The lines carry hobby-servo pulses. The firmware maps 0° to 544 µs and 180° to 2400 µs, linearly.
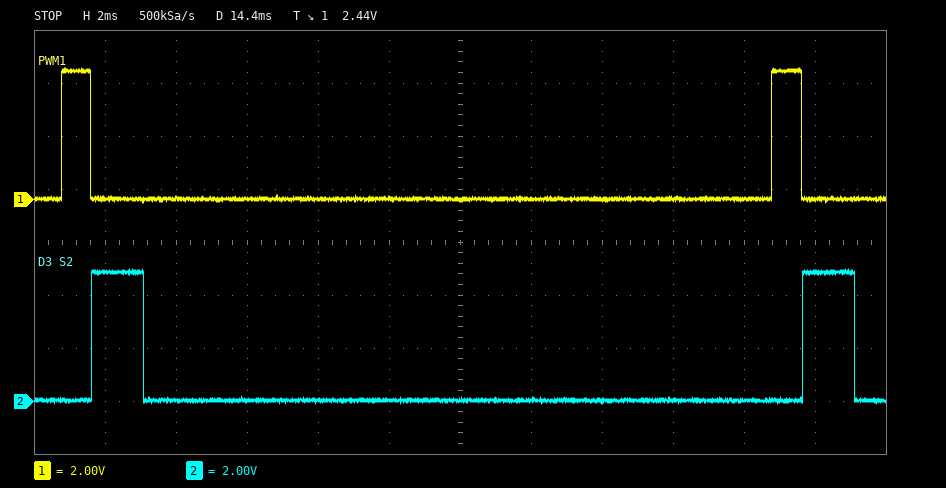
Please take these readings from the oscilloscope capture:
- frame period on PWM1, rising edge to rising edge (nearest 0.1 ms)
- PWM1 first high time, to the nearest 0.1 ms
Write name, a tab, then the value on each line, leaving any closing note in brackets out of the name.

frame period on PWM1, rising edge to rising edge	20.0 ms
PWM1 first high time, to the nearest 0.1 ms	0.8 ms
